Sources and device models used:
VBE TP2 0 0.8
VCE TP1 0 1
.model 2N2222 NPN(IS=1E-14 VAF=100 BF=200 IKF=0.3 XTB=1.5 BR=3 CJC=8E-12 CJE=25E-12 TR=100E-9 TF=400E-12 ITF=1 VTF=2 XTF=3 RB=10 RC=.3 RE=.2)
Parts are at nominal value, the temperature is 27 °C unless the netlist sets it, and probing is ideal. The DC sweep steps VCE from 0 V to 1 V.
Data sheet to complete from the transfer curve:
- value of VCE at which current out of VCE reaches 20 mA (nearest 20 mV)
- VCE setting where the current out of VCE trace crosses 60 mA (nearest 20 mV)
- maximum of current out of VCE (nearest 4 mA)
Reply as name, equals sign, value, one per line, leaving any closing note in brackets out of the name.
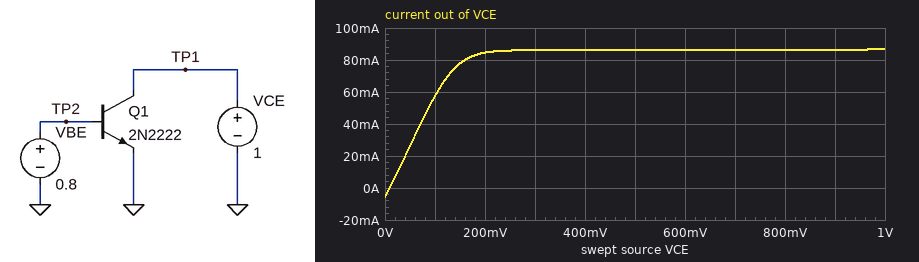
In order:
value of VCE at which current out of VCE reaches 20 mA = 40 mV
VCE setting where the current out of VCE trace crosses 60 mA = 100 mV
maximum of current out of VCE = 88 mA
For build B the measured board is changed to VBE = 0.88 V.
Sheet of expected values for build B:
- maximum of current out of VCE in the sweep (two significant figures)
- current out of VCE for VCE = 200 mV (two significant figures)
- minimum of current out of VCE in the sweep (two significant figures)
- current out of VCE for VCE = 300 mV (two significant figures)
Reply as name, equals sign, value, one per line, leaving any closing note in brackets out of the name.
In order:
maximum of current out of VCE in the sweep = 240 mA
current out of VCE for VCE = 200 mV = 190 mA
minimum of current out of VCE in the sweep = -9.6 mA
current out of VCE for VCE = 300 mV = 230 mA
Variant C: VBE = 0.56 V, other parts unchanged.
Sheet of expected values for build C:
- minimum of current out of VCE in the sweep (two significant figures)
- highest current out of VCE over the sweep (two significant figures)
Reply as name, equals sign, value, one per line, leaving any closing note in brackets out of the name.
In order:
minimum of current out of VCE in the sweep = -8.4 µA
highest current out of VCE over the sweep = 25 µA
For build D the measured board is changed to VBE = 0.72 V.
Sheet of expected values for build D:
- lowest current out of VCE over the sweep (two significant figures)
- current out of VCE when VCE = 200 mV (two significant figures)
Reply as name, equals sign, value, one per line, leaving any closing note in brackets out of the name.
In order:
lowest current out of VCE over the sweep = -1.8 mA
current out of VCE when VCE = 200 mV = 11 mA
